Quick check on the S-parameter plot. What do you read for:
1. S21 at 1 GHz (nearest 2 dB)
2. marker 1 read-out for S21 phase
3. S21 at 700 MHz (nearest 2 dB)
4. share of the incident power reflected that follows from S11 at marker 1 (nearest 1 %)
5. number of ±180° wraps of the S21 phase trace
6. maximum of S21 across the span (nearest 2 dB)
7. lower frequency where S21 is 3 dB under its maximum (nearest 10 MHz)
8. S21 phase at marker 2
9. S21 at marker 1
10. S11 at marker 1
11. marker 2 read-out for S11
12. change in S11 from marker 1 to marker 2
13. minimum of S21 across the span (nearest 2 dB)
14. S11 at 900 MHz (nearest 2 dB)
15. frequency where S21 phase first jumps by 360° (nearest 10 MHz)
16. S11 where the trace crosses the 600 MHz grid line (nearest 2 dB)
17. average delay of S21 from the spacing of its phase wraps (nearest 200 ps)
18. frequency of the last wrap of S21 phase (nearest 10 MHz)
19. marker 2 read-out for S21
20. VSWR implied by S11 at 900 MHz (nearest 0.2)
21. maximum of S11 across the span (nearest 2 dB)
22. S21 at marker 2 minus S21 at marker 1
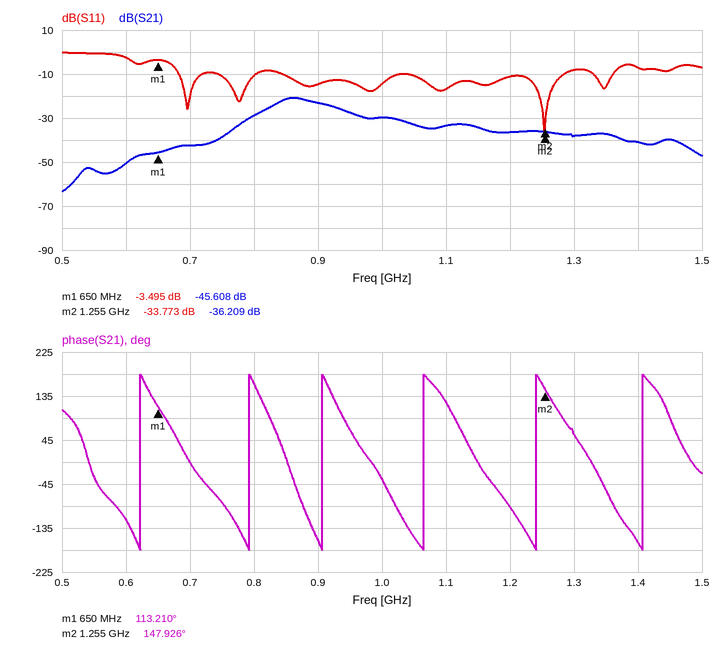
-30 dB
113.210°
-42 dB
45 %
6
-20 dB
830 MHz
147.926°
-45.608 dB
-3.495 dB
-33.773 dB
-30.278 dB
-64 dB
-14 dB
620 MHz
-2 dB
6.4 ns
1.41 GHz
-36.209 dB
1.4
0 dB
9.399 dB
